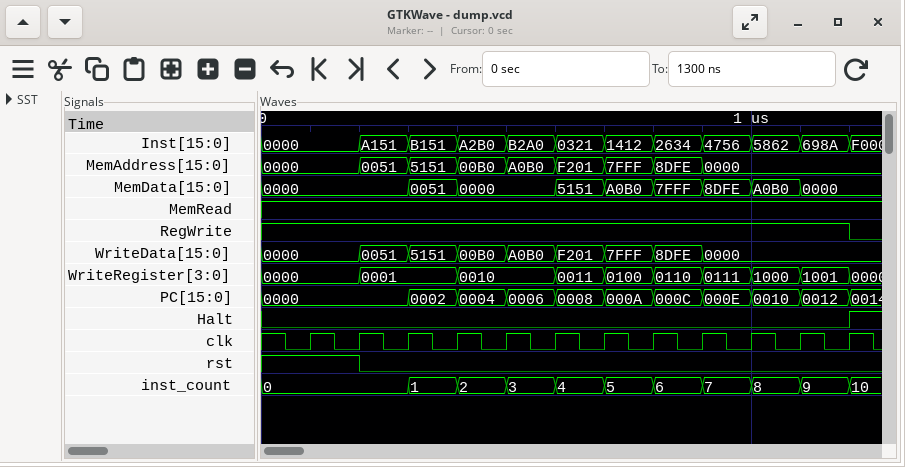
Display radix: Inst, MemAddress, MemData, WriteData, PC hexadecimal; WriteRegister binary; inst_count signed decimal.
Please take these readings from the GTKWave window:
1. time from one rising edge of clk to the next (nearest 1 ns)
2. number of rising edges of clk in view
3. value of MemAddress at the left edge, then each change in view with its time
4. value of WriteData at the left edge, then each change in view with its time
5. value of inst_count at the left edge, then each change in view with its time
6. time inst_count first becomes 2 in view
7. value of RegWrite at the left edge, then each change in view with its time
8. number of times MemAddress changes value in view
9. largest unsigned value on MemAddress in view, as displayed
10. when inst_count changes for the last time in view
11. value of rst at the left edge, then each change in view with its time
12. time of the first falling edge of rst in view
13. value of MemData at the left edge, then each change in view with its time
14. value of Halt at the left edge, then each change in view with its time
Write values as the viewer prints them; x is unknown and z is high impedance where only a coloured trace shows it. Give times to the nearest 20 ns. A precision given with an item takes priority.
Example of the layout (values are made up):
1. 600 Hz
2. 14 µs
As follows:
1. 100 ns
2. 12
3. 0000, 0051 at 200 ns, 5151 at 300 ns, 00B0 at 400 ns, A0B0 at 500 ns, F201 at 600 ns, 7FFF at 700 ns, 8DFE at 800 ns, 0000 at 900 ns
4. 0000, 0051 at 200 ns, 5151 at 300 ns, 00B0 at 400 ns, A0B0 at 500 ns, F201 at 600 ns, 7FFF at 700 ns, 8DFE at 800 ns, 0000 at 900 ns
5. 0, 1 at 300 ns, 2 at 400 ns, 3 at 500 ns, 4 at 600 ns, 5 at 700 ns, 6 at 800 ns, 7 at 900 ns, 8 at 1000 ns, 9 at 1100 ns, 10 at 1200 ns
6. 400 ns
7. 1, 0 at 1200 ns
8. 8
9. F201
10. 1200 ns
11. 1, 0 at 200 ns
12. 200 ns
13. 0000, 0051 at 300 ns, 0000 at 400 ns, 5151 at 600 ns, A0B0 at 700 ns, 7FFF at 800 ns, 8DFE at 900 ns, A0B0 at 1000 ns, 0000 at 1100 ns
14. 0, 1 at 1200 ns
